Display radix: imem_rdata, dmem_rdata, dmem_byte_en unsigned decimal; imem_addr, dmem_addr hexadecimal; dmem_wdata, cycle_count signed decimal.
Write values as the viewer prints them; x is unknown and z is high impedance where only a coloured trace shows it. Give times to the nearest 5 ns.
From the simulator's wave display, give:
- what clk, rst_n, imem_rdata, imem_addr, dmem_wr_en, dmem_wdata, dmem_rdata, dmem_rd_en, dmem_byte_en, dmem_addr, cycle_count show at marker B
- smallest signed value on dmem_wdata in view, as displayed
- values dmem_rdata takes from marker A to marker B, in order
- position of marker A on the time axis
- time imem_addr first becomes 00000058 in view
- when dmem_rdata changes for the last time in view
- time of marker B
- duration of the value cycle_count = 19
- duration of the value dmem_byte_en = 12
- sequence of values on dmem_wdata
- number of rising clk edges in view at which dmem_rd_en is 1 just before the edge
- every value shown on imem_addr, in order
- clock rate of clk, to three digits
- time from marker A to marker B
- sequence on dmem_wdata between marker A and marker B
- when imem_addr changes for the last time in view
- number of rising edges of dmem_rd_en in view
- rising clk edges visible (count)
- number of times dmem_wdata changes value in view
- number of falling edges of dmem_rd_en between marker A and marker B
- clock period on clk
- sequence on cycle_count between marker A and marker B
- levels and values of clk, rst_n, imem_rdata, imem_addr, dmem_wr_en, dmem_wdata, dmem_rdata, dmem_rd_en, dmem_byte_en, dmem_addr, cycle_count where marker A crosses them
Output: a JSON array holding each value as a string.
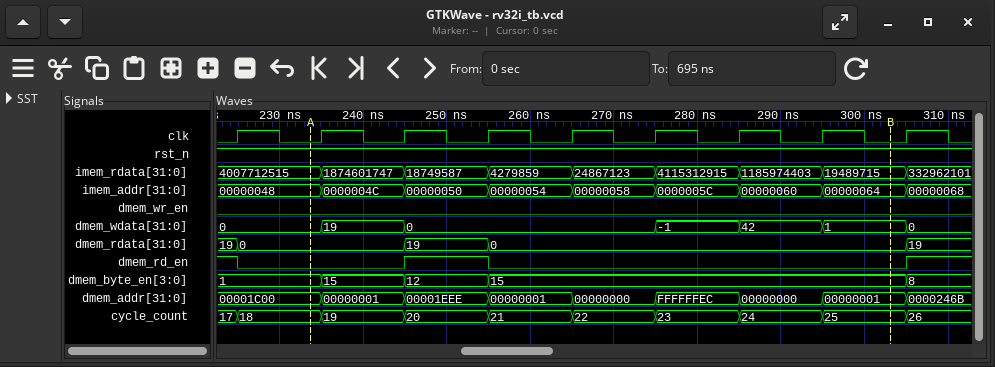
["clk=0, rst_n=1, imem_rdata=19489715, imem_addr=00000064, dmem_wr_en=0, dmem_wdata=1, dmem_rdata=0, dmem_rd_en=0, dmem_byte_en=15, dmem_addr=00000001, cycle_count=25", "-1", "0, 19, 0", "235 ns", "265 ns", "305 ns", "305 ns", "10 ns", "10 ns", "0, 19, 0, -1, 42, 1, 0", "2", "00000048, 0000004C, 00000050, 00000054, 00000058, 0000005C, 00000060, 00000064, 00000068", "100 MHz", "70 ns", "0, 19, 0, -1, 42, 1", "305 ns", "2", "9", "6", "1", "10 ns", "18, 19, 20, 21, 22, 23, 24, 25", "clk=0, rst_n=1, imem_rdata=4007712515, imem_addr=00000048, dmem_wr_en=0, dmem_wdata=0, dmem_rdata=0, dmem_rd_en=0, dmem_byte_en=1, dmem_addr=00001C00, cycle_count=18"]
